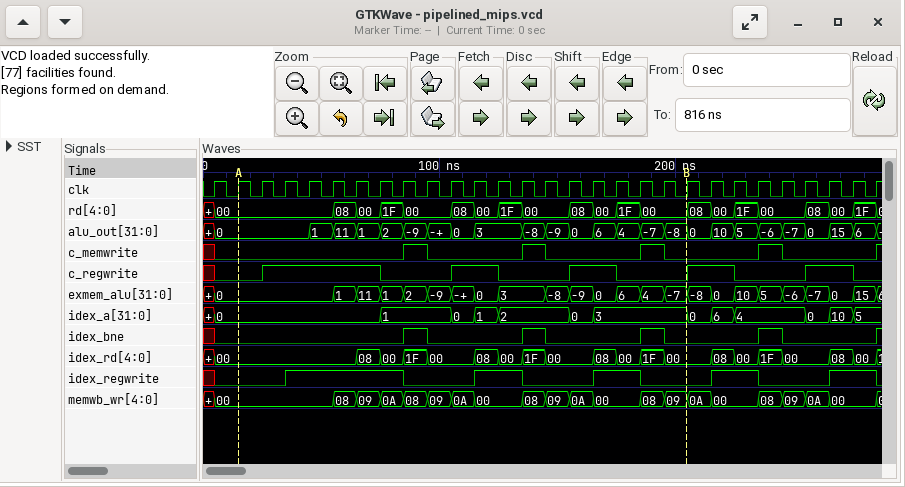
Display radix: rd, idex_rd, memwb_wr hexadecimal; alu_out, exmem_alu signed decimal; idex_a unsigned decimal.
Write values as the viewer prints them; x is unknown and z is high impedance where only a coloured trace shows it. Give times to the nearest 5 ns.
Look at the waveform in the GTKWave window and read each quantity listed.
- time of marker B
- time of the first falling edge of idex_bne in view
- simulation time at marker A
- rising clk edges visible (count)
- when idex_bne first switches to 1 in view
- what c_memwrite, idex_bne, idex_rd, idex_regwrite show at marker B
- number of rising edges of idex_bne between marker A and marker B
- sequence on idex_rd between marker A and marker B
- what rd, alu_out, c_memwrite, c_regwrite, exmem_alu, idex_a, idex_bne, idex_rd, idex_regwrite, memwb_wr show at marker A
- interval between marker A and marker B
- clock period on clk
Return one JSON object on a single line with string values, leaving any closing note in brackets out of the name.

{"time of marker B": "205 ns", "time of the first falling edge of idex_bne in view": "95 ns", "simulation time at marker A": "15 ns", "rising clk edges visible": "29", "when idex_bne first switches to 1 in view": "85 ns", "what c_memwrite, idex_bne, idex_rd, idex_regwrite show at marker B": "c_memwrite=0, idex_bne=0, idex_rd=00, idex_regwrite=0", "number of rising edges of idex_bne between marker A and marker B": "3", "sequence on idex_rd between marker A and marker B": "00, 08, 00, 1F, 00, 08, 00, 1F, 00, 08, 00, 1F, 00", "what rd, alu_out, c_memwrite, c_regwrite, exmem_alu, idex_a, idex_bne, idex_rd, idex_regwrite, memwb_wr show at marker A": "rd=00, alu_out=0, c_memwrite=0, c_regwrite=0, exmem_alu=0, idex_a=0, idex_bne=0, idex_rd=00, idex_regwrite=0, memwb_wr=00", "interval between marker A and marker B": "190 ns", "clock period on clk": "10 ns"}
